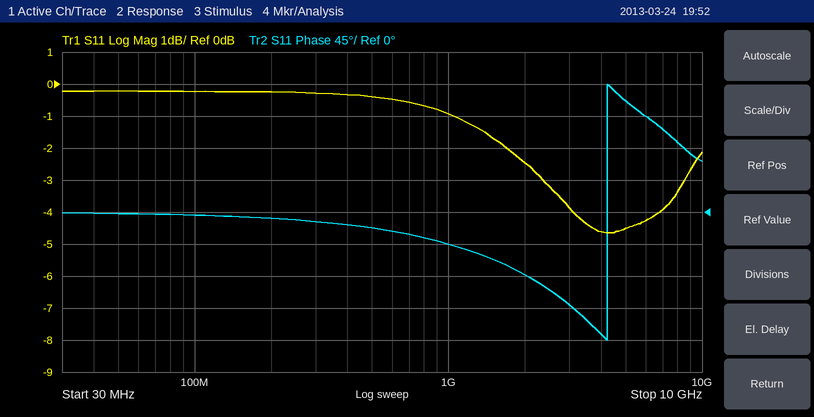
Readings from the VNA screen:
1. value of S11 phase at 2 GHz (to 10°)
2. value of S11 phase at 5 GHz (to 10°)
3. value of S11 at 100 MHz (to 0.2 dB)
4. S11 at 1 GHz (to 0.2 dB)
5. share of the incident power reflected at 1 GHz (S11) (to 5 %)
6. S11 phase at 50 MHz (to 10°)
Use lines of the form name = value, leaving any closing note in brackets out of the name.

value of S11 phase at 2 GHz = -90°
value of S11 phase at 5 GHz = 160°
value of S11 at 100 MHz = -0.2 dB
S11 at 1 GHz = -1.0 dB
share of the incident power reflected at 1 GHz (S11) = 80 %
S11 phase at 50 MHz = 0°
